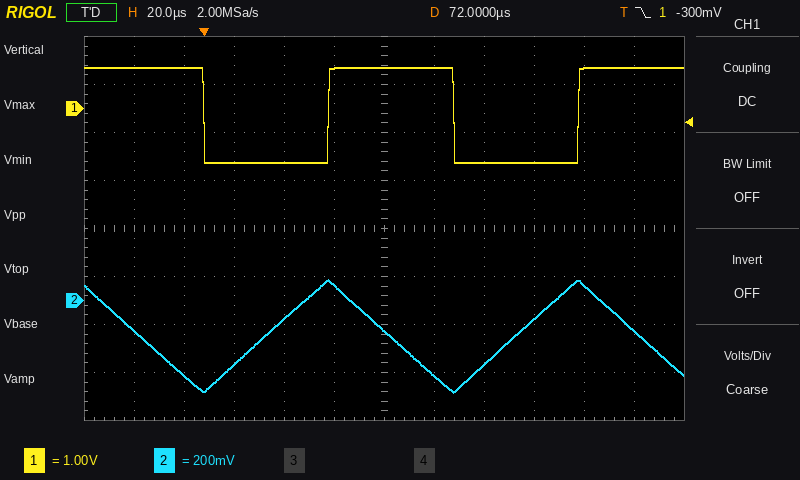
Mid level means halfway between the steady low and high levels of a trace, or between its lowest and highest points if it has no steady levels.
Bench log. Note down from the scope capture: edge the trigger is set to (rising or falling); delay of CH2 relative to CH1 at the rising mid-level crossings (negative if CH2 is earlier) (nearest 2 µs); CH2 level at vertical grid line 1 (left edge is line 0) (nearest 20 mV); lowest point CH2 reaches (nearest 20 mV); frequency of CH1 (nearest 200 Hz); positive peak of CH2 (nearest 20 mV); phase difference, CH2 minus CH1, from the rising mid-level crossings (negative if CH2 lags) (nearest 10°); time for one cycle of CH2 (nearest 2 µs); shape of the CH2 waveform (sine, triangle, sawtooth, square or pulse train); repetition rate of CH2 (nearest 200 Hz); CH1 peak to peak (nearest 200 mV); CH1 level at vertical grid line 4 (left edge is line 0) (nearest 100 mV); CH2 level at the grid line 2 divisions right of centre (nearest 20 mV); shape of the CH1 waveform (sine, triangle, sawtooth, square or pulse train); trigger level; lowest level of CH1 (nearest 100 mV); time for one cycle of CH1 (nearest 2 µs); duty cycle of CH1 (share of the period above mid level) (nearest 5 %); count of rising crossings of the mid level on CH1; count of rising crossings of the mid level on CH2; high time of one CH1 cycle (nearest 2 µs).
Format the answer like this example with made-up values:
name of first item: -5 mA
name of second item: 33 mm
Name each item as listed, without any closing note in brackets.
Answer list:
edge the trigger is set to: falling
delay of CH2 relative to CH1 at the rising mid-level crossings (negative if CH2 is earlier): -26 µs
CH2 level at vertical grid line 1 (left edge is line 0): -120 mV
lowest point CH2 reaches: -380 mV
frequency of CH1: 10.0 kHz
positive peak of CH2: 80 mV
phase difference, CH2 minus CH1, from the rising mid-level crossings (negative if CH2 lags): +90°
time for one cycle of CH2: 100 µs
shape of the CH2 waveform: triangle
repetition rate of CH2: 10.0 kHz
CH1 peak to peak: 2.0 V
CH1 level at vertical grid line 4 (left edge is line 0): -1.1 V
CH2 level at the grid line 2 divisions right of centre: -260 mV
shape of the CH1 waveform: square
trigger level: -300 mV
lowest level of CH1: -1.1 V
time for one cycle of CH1: 100 µs
duty cycle of CH1 (share of the period above mid level): 50 %
count of rising crossings of the mid level on CH1: 2
count of rising crossings of the mid level on CH2: 2
high time of one CH1 cycle: 50 µs
